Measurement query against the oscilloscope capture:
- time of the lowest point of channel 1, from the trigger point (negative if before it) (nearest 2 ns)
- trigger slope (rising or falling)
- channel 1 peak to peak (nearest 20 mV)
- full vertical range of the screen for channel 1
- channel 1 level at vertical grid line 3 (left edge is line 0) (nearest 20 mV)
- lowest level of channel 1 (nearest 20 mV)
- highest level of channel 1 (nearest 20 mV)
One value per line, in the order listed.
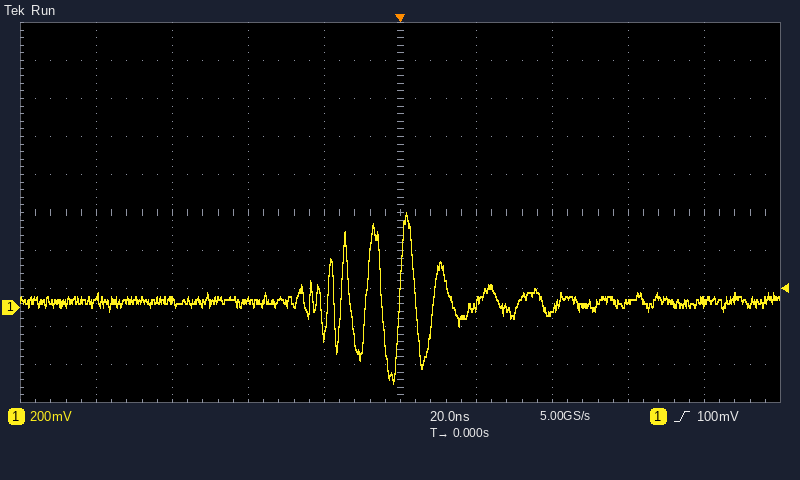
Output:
-2 ns
rising
900 mV
2 V
40 mV
-400 mV
500 mV
